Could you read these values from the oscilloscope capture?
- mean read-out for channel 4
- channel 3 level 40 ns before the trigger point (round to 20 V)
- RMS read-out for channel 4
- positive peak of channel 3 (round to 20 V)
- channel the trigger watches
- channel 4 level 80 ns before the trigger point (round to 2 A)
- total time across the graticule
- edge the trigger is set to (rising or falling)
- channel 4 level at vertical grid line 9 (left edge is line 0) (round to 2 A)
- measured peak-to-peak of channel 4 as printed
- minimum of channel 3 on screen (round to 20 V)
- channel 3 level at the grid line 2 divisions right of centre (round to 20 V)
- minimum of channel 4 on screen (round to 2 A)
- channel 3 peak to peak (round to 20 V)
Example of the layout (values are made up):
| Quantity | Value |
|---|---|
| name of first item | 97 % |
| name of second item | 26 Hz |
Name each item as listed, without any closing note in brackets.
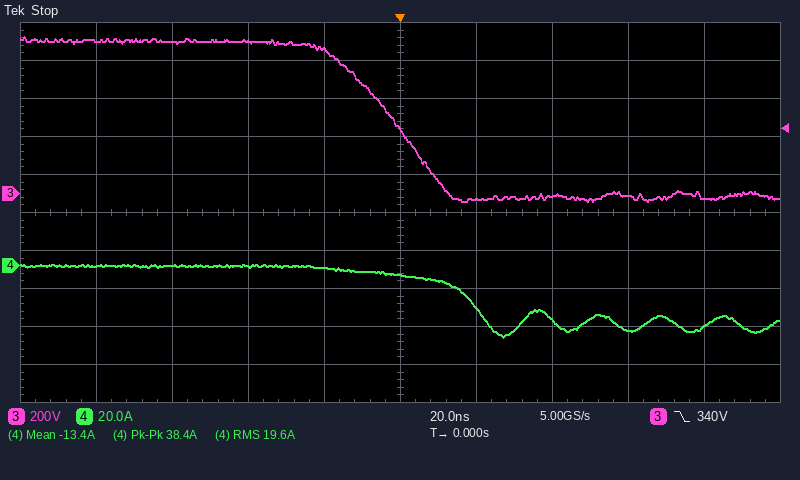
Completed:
| Quantity | Value |
|---|---|
| mean read-out for channel 4 | -13.4 A |
| channel 3 level 40 ns before the trigger point | 800 V |
| RMS read-out for channel 4 | 19.6 A |
| positive peak of channel 3 | 820 V |
| channel the trigger watches | channel 3 |
| channel 4 level 80 ns before the trigger point | 0 A |
| total time across the graticule | 200 ns |
| edge the trigger is set to | falling |
| channel 4 level at vertical grid line 9 (left edge is line 0) | -32 A |
| measured peak-to-peak of channel 4 as printed | 38.4 A |
| minimum of channel 3 on screen | -40 V |
| channel 3 level at the grid line 2 divisions right of centre | -20 V |
| minimum of channel 4 on screen | -38 A |
| channel 3 peak to peak | 860 V |
